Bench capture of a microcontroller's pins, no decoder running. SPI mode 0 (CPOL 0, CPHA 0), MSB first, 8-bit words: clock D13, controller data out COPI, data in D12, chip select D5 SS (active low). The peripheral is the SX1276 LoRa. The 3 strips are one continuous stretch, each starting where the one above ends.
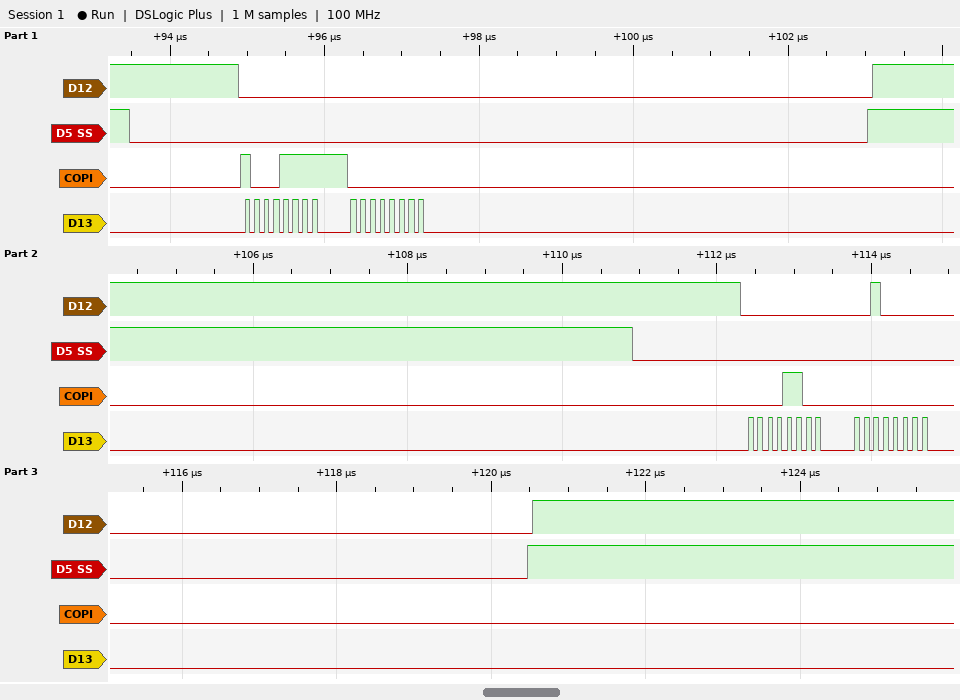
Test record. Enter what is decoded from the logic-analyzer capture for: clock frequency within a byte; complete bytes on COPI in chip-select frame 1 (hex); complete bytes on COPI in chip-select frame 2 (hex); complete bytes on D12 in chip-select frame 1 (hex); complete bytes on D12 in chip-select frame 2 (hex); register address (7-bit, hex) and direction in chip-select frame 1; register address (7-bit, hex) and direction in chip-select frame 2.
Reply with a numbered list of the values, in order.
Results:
1. 8 MHz
2. 8F 00
3. 0C 00
4. 00 00
5. 00 20
6. 0x0F write
7. 0x0C read
